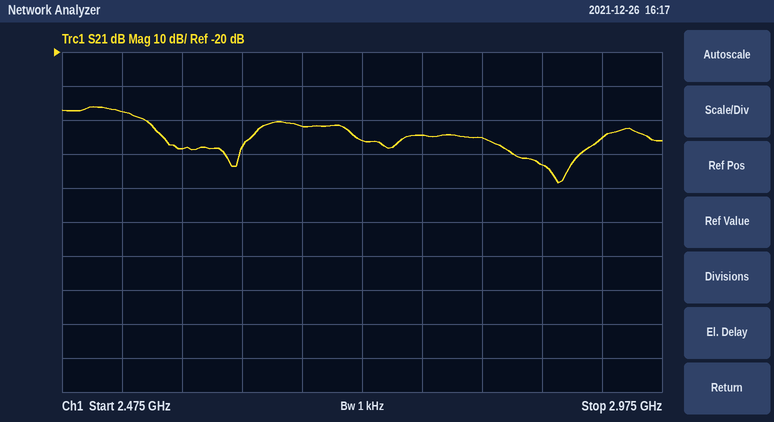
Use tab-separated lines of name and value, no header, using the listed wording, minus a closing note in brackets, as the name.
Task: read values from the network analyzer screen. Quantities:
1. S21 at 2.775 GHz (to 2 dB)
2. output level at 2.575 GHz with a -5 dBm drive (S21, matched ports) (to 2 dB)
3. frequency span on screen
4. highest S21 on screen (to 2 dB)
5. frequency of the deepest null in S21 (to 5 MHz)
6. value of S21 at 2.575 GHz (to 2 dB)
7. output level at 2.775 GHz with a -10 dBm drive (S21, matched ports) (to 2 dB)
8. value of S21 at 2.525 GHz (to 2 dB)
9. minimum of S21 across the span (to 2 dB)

S21 at 2.775 GHz	-44 dB
output level at 2.575 GHz with a -5 dBm drive (S21, matched ports)	-54 dBm
frequency span on screen	500 MHz
highest S21 on screen	-36 dB
frequency of the deepest null in S21	2.890 GHz
value of S21 at 2.575 GHz	-48 dB
output level at 2.775 GHz with a -10 dBm drive (S21, matched ports)	-54 dBm
value of S21 at 2.525 GHz	-38 dB
minimum of S21 across the span	-58 dB
